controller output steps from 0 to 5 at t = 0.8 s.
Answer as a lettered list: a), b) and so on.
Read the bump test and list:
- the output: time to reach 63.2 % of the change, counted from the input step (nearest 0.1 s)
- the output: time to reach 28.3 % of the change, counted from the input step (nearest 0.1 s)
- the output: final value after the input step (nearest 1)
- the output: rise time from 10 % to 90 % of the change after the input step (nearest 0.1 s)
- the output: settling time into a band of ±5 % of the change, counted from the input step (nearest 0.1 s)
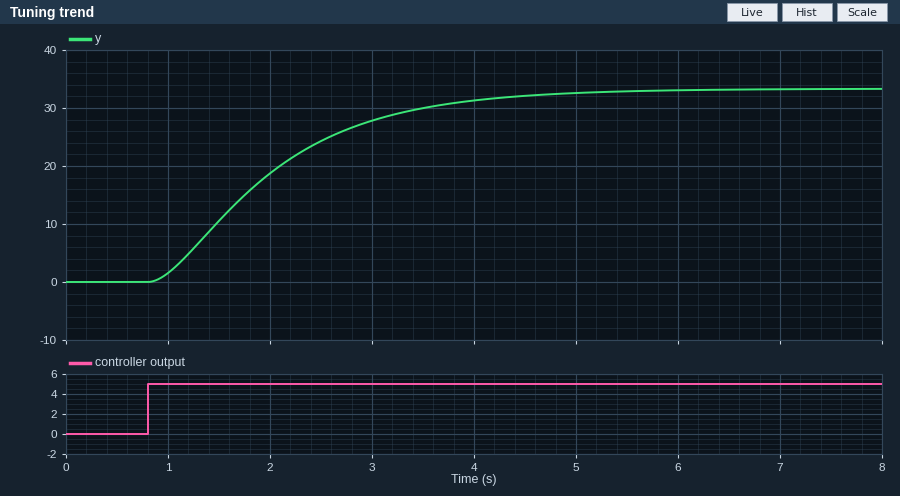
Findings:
a) 1.4 s
b) 0.6 s
c) 33
d) 2.4 s
e) 3.4 s
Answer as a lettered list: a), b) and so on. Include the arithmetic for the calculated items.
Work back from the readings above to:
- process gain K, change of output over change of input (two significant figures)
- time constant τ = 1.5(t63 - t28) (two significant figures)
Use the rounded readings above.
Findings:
a) (33 - 0) / 5 = 6.6
b) 1.5 × (1.4 - 0.6) = 1.2 s
